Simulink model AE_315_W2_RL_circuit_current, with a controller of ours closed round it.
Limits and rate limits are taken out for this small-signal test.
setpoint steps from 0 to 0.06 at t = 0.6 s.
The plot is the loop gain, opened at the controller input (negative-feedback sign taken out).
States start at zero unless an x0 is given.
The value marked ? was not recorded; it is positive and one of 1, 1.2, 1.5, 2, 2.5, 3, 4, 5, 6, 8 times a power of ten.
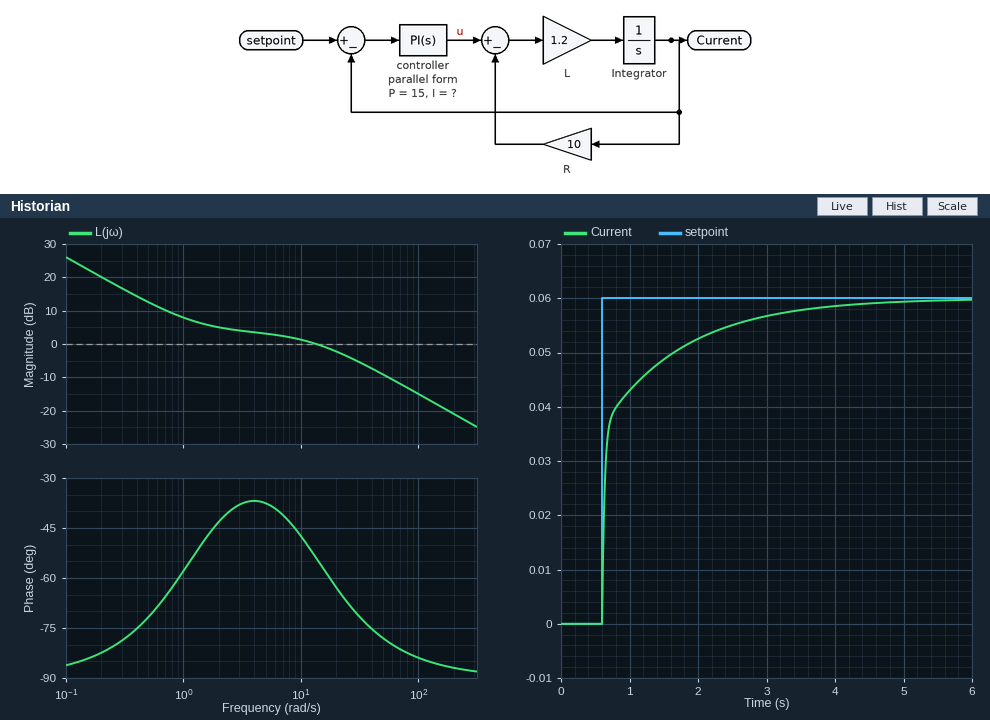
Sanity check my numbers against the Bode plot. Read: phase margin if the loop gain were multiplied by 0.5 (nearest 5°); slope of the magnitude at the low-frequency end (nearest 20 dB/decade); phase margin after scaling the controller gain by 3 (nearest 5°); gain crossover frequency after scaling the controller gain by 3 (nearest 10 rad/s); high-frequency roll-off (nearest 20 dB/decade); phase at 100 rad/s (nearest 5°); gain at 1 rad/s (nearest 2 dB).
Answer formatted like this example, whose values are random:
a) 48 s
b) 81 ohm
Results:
a) 130°
b) -20 dB/decade
c) 100°
d) 50 rad/s
e) -20 dB/decade
f) -85°
g) 8 dB
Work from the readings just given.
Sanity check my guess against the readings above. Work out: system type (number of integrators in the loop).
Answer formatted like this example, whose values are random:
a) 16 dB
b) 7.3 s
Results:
a) 1
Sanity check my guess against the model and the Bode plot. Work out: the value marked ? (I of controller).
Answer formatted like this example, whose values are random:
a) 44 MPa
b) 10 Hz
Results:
a) 20
